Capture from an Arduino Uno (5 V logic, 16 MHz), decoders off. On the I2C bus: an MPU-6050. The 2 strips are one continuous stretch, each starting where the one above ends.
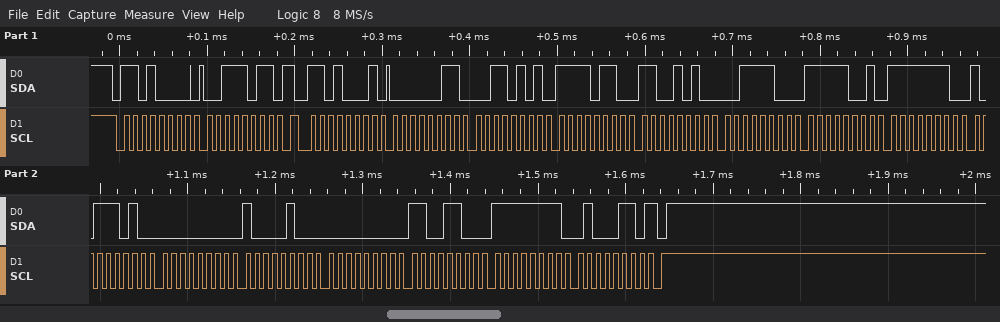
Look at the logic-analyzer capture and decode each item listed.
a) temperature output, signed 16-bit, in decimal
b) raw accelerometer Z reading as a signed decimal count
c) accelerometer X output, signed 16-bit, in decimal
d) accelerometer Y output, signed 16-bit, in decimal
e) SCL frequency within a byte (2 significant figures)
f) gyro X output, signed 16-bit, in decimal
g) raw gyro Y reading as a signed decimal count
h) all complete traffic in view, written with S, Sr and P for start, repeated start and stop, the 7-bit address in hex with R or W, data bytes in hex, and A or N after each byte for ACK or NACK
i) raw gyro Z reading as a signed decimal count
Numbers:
-326
15609
821
-2358
100 kHz
132
204
S 68W A 3B A Sr 68R A 03 A 35 A F6 A CA A 3C A F9 A FE A BA A 00 A 84 A 00 A CC A FF A 46 N P
-186
